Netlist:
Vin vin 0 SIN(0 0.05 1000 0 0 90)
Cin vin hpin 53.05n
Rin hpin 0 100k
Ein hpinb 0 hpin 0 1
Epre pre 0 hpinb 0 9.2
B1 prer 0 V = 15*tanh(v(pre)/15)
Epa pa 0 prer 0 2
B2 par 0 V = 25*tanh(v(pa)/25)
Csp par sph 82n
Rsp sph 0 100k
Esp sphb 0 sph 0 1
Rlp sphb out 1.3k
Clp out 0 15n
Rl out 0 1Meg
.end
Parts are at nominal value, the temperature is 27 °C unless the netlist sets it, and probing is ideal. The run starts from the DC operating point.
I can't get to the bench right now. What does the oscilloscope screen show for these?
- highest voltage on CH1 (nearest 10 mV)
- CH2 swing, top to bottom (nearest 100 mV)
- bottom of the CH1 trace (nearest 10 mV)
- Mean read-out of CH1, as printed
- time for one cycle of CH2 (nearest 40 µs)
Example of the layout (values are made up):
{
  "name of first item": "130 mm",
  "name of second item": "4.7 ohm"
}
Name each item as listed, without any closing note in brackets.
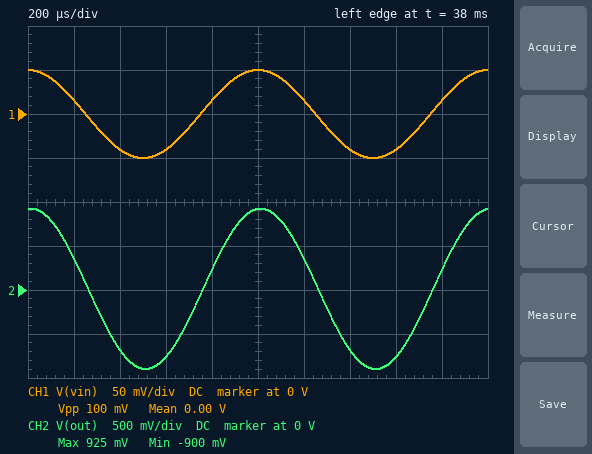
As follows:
{
  "highest voltage on CH1": "50 mV",
  "CH2 swing, top to bottom": "1.8 V",
  "bottom of the CH1 trace": "-50 mV",
  "Mean read-out of CH1, as printed": "0.00 V",
  "time for one cycle of CH2": "1.00 ms"
}
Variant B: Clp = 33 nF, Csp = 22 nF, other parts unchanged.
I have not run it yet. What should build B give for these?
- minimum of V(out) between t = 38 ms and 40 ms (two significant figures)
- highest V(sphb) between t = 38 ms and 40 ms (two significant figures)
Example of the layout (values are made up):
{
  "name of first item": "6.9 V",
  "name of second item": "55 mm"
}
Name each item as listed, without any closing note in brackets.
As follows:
{
  "minimum of V(out) between t = 38 ms and 40 ms": "-880 mV",
  "highest V(sphb) between t = 38 ms and 40 ms": "920 mV"
}
